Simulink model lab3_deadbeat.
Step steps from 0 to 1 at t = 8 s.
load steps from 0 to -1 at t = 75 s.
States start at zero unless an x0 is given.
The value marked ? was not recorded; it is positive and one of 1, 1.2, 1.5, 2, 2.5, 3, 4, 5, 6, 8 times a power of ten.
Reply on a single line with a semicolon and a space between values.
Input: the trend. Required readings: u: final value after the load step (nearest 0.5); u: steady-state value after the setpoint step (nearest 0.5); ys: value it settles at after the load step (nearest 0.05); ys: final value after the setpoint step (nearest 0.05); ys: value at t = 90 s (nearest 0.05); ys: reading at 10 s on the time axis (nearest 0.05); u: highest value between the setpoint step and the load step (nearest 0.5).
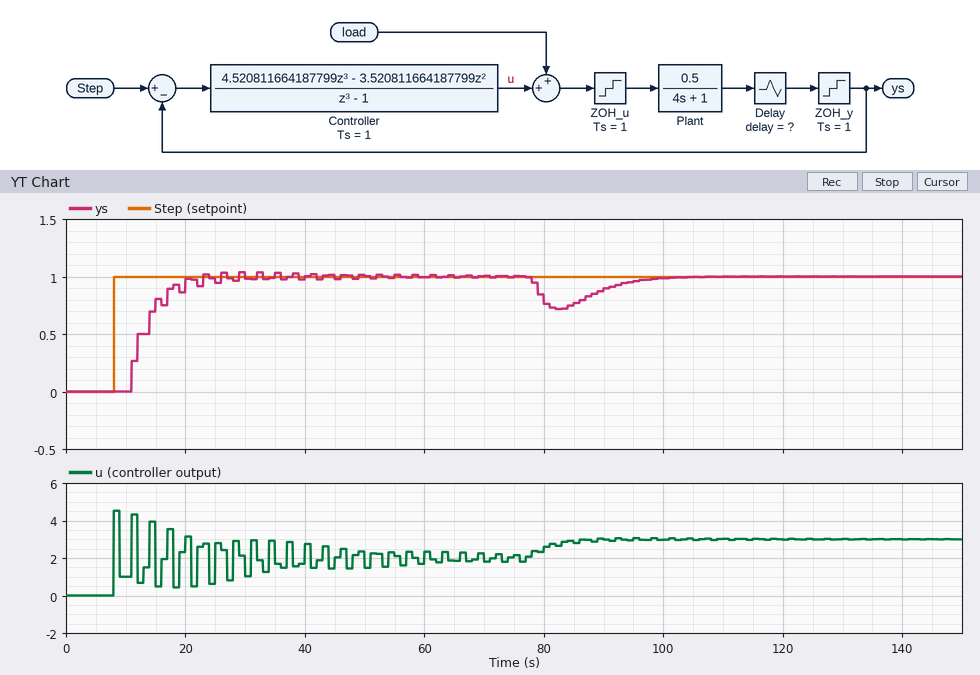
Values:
3.0; 2.0; 1.00; 1.00; 0.90; 0.00; 4.5
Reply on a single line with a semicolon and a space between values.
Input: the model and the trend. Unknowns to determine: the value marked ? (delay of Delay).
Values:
2.5
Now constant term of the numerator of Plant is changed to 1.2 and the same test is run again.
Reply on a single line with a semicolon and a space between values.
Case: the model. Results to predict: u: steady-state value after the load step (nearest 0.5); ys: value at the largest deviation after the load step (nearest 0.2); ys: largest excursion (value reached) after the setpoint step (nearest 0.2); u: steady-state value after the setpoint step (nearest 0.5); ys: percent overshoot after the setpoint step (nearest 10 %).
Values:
2.0; 0.4; 1.4; 1.0; 40 %
